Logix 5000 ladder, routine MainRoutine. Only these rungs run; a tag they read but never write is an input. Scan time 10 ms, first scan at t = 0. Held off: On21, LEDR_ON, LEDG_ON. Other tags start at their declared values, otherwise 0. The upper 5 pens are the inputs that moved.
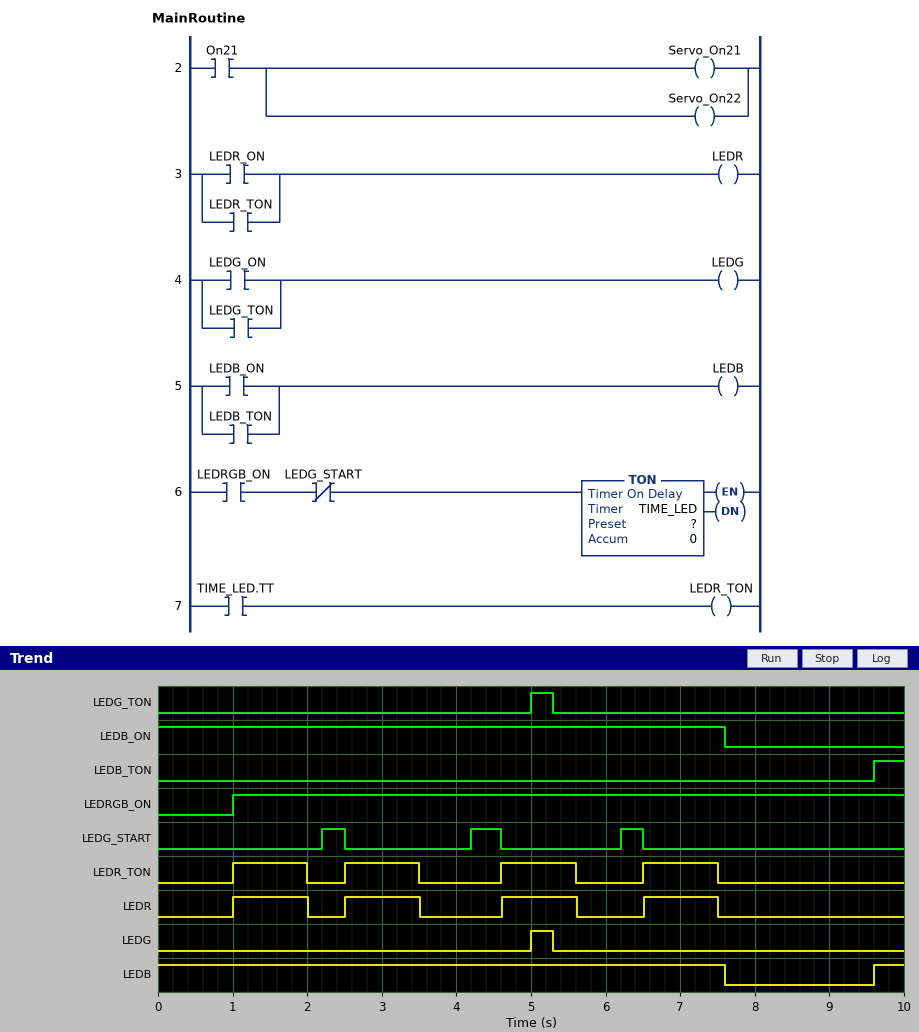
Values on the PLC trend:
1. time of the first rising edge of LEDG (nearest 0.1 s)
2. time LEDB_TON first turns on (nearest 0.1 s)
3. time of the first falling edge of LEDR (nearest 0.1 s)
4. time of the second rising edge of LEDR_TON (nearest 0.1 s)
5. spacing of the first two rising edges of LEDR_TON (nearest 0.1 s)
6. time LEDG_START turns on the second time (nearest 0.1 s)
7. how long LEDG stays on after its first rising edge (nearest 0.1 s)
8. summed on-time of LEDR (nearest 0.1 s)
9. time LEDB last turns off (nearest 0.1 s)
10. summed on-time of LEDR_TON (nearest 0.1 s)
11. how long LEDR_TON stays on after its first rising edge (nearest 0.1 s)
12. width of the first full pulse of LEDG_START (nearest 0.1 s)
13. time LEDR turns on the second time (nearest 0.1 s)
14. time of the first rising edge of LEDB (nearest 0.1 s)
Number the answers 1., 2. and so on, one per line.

1. 5.0 s
2. 9.6 s
3. 2.0 s
4. 2.5 s
5. 1.5 s
6. 4.2 s
7. 0.3 s
8. 4.0 s
9. 7.6 s
10. 4.0 s
11. 1.0 s
12. 0.3 s
13. 2.5 s
14. 9.6 s
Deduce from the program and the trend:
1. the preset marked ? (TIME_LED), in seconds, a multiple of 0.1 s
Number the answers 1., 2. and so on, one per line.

1. 1.0 s
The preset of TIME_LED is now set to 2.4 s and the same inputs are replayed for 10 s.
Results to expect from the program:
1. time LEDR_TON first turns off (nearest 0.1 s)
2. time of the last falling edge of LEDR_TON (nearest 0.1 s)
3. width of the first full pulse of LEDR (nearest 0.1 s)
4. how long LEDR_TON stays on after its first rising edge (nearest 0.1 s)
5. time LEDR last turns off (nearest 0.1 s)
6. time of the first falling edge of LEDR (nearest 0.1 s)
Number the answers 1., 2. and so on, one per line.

1. 2.2 s
2. 8.9 s
3. 1.2 s
4. 1.2 s
5. 8.9 s
6. 2.2 s
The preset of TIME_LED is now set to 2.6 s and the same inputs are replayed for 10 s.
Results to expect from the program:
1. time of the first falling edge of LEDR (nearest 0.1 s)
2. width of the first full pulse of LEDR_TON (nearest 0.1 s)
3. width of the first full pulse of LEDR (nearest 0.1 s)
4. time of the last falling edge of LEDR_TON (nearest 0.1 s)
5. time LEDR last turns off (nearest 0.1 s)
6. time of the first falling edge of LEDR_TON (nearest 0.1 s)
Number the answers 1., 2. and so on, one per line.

1. 2.2 s
2. 1.2 s
3. 1.2 s
4. 9.1 s
5. 9.1 s
6. 2.2 s
